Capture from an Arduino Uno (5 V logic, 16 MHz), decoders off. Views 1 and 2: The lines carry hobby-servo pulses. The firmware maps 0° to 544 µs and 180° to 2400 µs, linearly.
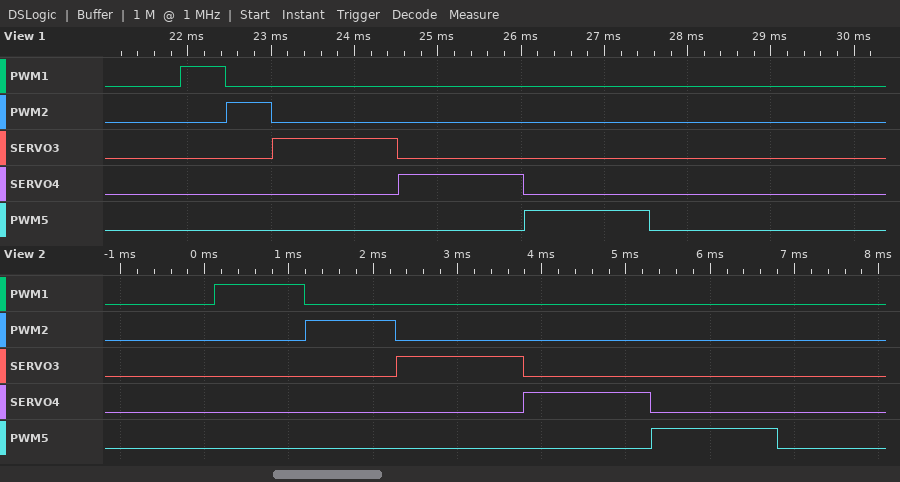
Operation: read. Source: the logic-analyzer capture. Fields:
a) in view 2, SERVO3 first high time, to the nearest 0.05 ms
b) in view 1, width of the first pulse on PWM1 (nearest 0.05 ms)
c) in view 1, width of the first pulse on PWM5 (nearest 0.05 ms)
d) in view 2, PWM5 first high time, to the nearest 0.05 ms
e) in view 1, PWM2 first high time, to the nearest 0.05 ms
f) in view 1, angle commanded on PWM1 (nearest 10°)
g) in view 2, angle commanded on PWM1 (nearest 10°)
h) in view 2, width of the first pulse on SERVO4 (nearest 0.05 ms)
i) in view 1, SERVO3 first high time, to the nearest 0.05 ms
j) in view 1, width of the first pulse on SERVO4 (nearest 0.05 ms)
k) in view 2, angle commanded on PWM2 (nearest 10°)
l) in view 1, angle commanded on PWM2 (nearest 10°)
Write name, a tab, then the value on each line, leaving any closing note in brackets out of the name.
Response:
in view 2, SERVO3 first high time, to the nearest 0.05 ms	1.50 ms
in view 1, width of the first pulse on PWM1	0.55 ms
in view 1, width of the first pulse on PWM5	1.50 ms
in view 2, PWM5 first high time, to the nearest 0.05 ms	1.50 ms
in view 1, PWM2 first high time, to the nearest 0.05 ms	0.55 ms
in view 1, angle commanded on PWM1	0°
in view 2, angle commanded on PWM1	50°
in view 2, width of the first pulse on SERVO4	1.50 ms
in view 1, SERVO3 first high time, to the nearest 0.05 ms	1.50 ms
in view 1, width of the first pulse on SERVO4	1.50 ms
in view 2, angle commanded on PWM2	50°
in view 1, angle commanded on PWM2	0°
